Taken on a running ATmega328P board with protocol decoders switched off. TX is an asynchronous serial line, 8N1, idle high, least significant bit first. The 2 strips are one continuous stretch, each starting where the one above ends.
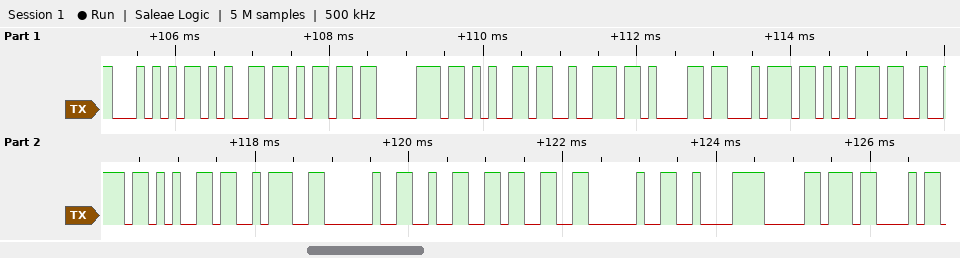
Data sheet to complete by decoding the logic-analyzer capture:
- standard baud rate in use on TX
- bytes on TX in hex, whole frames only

9600 baud
54 65 6D 70 65 72 61 74 75 72 65 3A 20 32 33 20 C2 B0 43
